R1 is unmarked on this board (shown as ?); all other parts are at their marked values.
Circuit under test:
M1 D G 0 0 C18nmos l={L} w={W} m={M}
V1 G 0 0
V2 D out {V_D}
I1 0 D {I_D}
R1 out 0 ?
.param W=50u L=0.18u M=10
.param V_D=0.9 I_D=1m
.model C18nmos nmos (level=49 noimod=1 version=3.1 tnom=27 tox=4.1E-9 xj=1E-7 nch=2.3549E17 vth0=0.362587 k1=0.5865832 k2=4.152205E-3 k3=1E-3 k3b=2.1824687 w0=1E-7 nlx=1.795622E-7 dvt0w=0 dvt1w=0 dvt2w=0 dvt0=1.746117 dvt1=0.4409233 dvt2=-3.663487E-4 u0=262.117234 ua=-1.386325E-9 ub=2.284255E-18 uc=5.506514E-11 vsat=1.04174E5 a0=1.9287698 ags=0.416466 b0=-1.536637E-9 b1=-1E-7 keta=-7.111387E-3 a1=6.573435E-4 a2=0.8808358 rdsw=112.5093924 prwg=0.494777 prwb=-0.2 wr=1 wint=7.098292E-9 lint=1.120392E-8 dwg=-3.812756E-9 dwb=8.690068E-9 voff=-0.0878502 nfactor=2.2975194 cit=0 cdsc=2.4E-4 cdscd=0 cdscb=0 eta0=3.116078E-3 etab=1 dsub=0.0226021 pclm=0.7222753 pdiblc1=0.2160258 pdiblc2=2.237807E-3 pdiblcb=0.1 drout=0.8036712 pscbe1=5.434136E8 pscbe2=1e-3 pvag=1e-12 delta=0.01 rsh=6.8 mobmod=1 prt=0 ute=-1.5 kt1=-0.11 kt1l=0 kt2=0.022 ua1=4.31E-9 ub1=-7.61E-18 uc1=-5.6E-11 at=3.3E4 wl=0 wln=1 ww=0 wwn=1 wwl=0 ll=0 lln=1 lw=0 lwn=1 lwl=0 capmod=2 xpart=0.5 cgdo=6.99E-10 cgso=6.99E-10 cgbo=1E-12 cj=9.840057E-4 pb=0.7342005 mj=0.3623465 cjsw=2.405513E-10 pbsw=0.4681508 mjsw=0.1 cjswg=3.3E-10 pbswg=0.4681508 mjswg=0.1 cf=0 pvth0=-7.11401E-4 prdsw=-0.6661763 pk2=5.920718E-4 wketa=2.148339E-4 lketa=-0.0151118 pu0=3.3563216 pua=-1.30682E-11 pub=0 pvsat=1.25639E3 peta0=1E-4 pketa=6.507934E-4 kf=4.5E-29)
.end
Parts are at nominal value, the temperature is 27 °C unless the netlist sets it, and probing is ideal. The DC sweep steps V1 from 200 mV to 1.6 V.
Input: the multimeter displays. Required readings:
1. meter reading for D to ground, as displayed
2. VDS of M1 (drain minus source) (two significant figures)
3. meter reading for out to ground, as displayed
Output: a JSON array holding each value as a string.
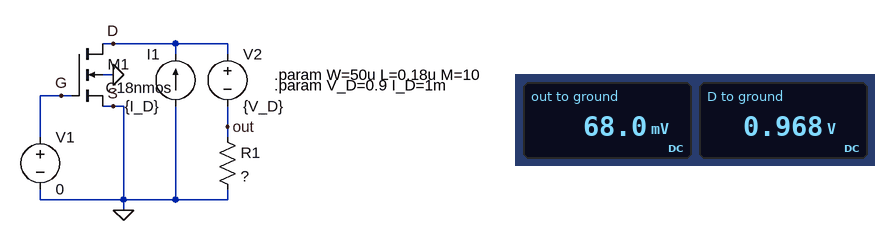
["0.968 V", "970 mV", "68.0 mV"]
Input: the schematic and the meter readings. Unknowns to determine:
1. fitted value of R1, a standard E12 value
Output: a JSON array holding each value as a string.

["68 Ω"]
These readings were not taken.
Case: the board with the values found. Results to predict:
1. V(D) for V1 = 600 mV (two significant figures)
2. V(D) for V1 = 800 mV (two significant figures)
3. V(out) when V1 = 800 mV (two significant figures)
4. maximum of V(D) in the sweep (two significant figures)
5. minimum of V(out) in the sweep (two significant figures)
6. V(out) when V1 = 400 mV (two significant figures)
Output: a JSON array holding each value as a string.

["600 mV", "83 mV", "-820 mV", "970 mV", "-860 mV", "59 mV"]
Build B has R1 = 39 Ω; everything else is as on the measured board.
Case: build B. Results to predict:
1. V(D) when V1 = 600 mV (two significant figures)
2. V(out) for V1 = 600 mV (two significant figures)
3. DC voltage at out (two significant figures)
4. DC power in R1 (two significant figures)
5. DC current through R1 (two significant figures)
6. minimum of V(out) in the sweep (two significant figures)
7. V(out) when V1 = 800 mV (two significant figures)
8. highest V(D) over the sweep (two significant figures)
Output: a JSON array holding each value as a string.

["720 mV", "-180 mV", "39 mV", "39 µW", "1.0 mA", "-830 mV", "-750 mV", "940 mV"]
